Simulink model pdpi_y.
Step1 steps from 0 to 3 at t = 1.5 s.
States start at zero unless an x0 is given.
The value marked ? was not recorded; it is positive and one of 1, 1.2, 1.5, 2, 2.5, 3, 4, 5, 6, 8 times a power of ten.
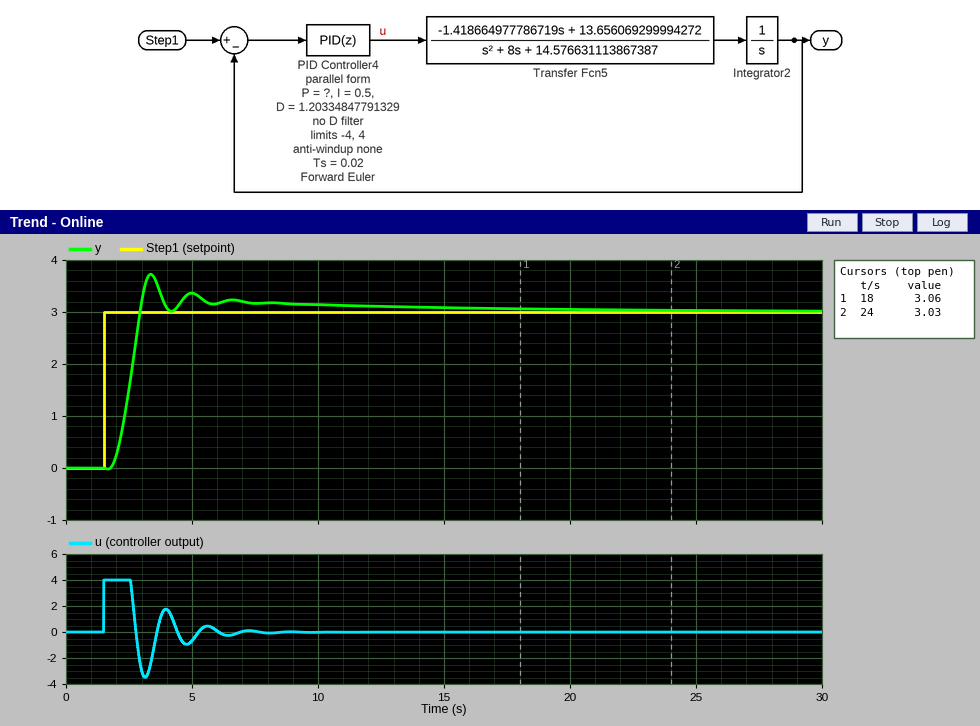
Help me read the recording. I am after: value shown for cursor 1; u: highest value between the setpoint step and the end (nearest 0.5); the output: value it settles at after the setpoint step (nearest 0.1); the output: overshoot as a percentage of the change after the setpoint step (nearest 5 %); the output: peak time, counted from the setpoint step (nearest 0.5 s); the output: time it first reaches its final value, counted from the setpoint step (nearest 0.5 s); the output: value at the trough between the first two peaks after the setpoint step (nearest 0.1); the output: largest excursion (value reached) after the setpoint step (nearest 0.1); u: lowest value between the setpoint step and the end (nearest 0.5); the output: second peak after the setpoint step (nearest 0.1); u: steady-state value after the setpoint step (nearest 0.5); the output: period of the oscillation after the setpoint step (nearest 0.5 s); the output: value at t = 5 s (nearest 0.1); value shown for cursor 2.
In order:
3.06
4.0
3.0
25 %
2.0 s
1.5 s
3.0
3.7
-3.5
3.4
0.0
1.5 s
3.4
3.03
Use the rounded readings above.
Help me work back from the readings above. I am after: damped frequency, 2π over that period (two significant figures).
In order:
4.2 rad/s
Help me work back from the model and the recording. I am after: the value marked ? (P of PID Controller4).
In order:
5
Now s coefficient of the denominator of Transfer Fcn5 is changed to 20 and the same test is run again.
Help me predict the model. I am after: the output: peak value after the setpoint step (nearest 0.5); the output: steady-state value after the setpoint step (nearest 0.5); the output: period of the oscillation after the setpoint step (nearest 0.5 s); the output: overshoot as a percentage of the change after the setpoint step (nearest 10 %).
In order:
4.0
3.0
3.5 s
40 %
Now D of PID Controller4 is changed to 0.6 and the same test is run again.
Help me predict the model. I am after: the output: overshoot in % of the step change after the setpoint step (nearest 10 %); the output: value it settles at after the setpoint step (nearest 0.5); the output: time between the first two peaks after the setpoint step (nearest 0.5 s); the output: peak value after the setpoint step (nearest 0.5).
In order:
40 %
3.0
2.0 s
4.0
